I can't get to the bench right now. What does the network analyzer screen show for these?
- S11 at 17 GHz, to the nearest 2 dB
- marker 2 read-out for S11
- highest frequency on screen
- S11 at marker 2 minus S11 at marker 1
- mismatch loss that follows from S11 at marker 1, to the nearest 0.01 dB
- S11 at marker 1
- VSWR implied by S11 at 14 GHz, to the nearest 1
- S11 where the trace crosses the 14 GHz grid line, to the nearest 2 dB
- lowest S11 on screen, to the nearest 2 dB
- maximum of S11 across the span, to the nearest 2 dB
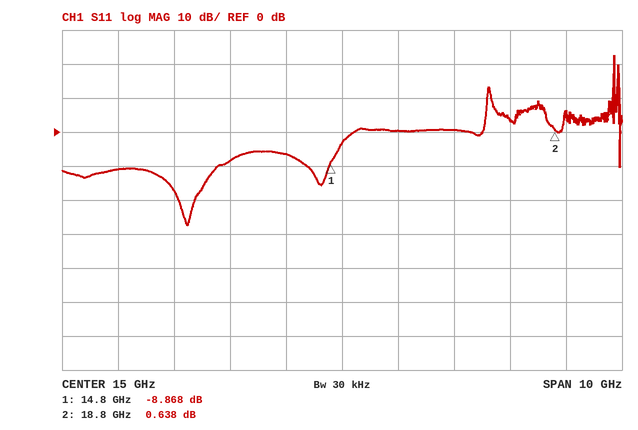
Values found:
0 dB
0.638 dB
20 GHz
9.506 dB
0.60 dB
-8.868 dB
3
-6 dB
-28 dB
22 dB
